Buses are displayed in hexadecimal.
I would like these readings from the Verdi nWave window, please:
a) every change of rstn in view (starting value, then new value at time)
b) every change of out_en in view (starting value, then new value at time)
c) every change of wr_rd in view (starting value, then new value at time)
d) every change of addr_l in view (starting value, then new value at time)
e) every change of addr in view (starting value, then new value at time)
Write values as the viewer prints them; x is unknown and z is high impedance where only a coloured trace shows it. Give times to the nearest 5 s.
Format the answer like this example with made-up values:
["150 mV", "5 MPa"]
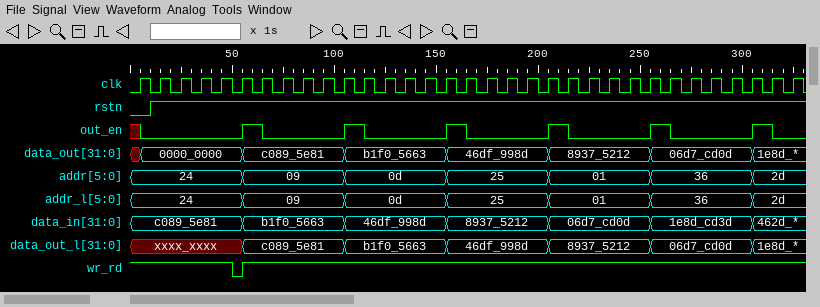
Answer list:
["0, 1 at 10 s", "x, 0 at 5 s, 1 at 55 s, 0 at 65 s, 1 at 105 s, 0 at 115 s, 1 at 155 s, 0 at 165 s, 1 at 205 s, 0 at 215 s, 1 at 255 s, 0 at 265 s, 1 at 305 s, 0 at 315 s", "1, 0 at 50 s, 1 at 55 s", "24, 09 at 55 s, 0d at 105 s, 25 at 155 s, 01 at 205 s, 36 at 255 s, 2d at 305 s", "24, 09 at 55 s, 0d at 105 s, 25 at 155 s, 01 at 205 s, 36 at 255 s, 2d at 305 s"]
